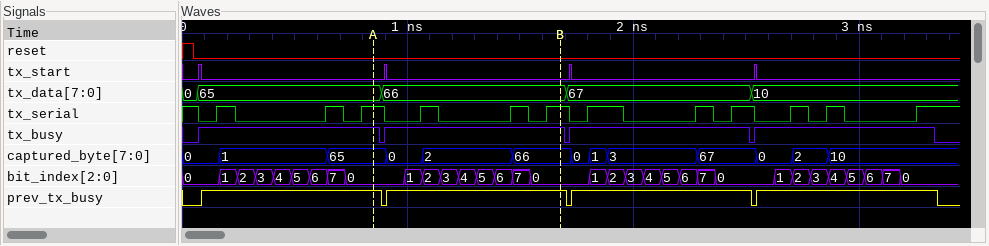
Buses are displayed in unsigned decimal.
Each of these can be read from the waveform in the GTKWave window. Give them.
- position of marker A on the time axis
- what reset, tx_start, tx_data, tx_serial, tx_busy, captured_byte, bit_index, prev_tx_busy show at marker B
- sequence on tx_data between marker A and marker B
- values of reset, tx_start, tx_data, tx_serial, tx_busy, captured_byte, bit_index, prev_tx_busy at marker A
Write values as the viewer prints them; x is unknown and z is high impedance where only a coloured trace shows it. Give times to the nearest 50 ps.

850 ps
reset=0, tx_start=0, tx_data=66, tx_serial=1, tx_busy=1, captured_byte=66, bit_index=0, prev_tx_busy=1
65, 66
reset=0, tx_start=0, tx_data=65, tx_serial=1, tx_busy=1, captured_byte=65, bit_index=0, prev_tx_busy=1
